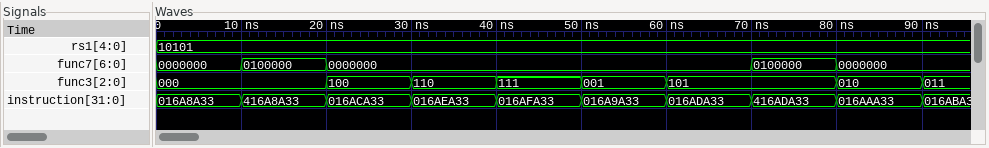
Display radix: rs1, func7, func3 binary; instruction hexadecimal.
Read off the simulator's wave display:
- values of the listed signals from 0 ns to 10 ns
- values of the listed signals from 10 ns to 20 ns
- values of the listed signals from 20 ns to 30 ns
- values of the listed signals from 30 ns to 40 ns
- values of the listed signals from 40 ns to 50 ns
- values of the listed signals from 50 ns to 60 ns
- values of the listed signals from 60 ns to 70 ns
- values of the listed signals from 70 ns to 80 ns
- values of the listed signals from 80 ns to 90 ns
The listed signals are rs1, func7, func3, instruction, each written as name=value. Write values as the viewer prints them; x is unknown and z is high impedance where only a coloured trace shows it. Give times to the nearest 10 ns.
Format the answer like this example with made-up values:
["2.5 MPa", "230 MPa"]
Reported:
["rs1=10101, func7=0000000, func3=000, instruction=016A8A33", "rs1=10101, func7=0100000, func3=000, instruction=416A8A33", "rs1=10101, func7=0000000, func3=100, instruction=016ACA33", "rs1=10101, func7=0000000, func3=110, instruction=016AEA33", "rs1=10101, func7=0000000, func3=111, instruction=016AFA33", "rs1=10101, func7=0000000, func3=001, instruction=016A9A33", "rs1=10101, func7=0000000, func3=101, instruction=016ADA33", "rs1=10101, func7=0100000, func3=101, instruction=416ADA33", "rs1=10101, func7=0000000, func3=010, instruction=016AAA33"]
